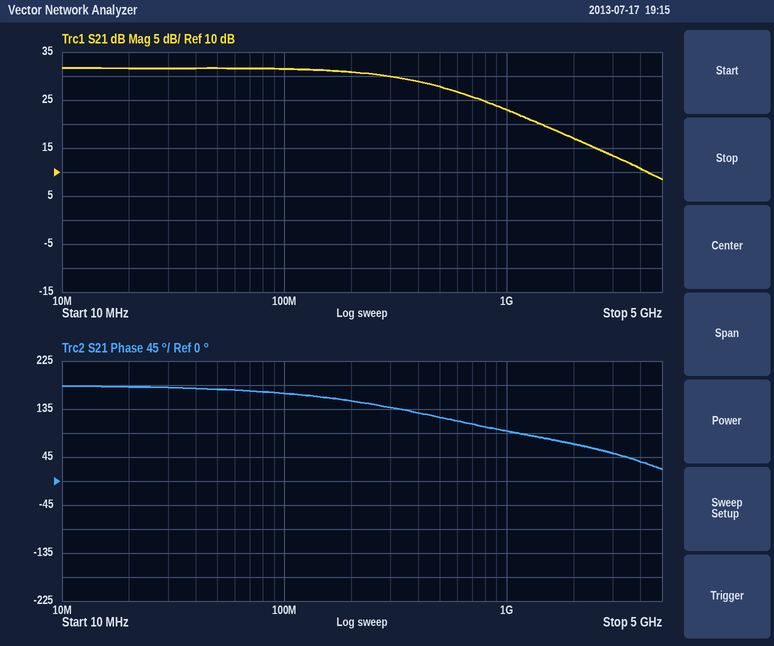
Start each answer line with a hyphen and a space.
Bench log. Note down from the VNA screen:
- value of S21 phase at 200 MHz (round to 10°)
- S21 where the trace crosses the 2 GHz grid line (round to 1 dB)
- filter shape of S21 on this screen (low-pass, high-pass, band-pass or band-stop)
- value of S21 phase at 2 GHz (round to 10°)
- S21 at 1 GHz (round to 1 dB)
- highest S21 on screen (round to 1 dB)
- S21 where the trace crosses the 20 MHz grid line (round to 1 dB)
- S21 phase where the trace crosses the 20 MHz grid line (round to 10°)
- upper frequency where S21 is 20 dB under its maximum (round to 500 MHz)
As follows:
- 150°
- 17 dB
- low-pass
- 70°
- 23 dB
- 32 dB
- 32 dB
- 180°
- 3.5 GHz
